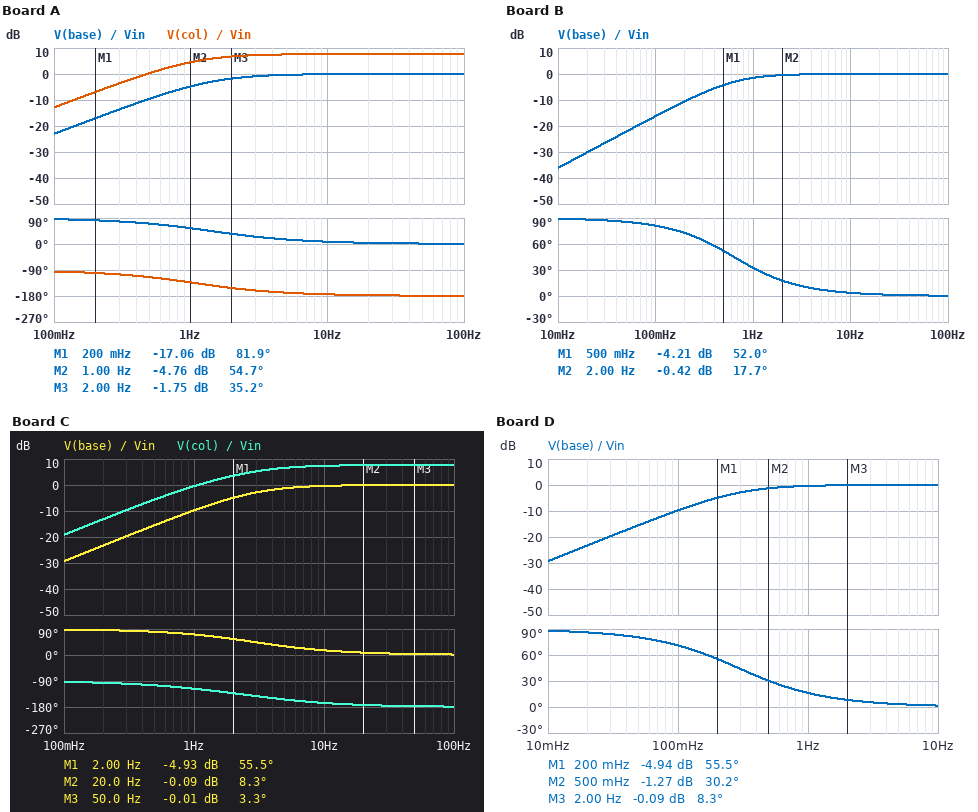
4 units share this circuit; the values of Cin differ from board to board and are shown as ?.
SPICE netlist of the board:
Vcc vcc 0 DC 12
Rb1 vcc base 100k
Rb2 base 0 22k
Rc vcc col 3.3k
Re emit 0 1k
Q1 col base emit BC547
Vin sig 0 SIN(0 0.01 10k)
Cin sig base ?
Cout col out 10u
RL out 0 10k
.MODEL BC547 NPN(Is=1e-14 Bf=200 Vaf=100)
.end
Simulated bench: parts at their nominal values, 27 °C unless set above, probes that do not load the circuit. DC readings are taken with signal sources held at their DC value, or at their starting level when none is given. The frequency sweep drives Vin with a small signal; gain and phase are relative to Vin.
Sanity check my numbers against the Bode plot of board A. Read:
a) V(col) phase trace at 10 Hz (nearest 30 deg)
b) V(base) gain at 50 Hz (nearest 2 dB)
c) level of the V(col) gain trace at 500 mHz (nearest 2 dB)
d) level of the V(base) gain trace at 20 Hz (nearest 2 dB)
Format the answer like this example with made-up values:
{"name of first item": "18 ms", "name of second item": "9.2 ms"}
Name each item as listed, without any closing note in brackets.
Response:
{"V(col) phase trace at 10 Hz": "-180 deg", "V(base) gain at 50 Hz": "0 dB", "level of the V(col) gain trace at 500 mHz": "0 dB", "level of the V(base) gain trace at 20 Hz": "0 dB"}
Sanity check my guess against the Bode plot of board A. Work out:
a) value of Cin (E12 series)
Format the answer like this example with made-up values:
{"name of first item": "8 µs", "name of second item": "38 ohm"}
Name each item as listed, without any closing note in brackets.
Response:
{"value of Cin": "6.8 µF"}
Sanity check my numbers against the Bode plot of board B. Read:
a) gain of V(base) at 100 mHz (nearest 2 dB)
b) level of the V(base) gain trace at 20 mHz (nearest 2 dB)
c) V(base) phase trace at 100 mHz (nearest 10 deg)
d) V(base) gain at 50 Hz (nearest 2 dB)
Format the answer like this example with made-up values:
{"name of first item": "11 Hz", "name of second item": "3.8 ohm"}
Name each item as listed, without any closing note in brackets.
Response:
{"gain of V(base) at 100 mHz": "-16 dB", "level of the V(base) gain trace at 20 mHz": "-30 dB", "V(base) phase trace at 100 mHz": "80 deg", "V(base) gain at 50 Hz": "0 dB"}
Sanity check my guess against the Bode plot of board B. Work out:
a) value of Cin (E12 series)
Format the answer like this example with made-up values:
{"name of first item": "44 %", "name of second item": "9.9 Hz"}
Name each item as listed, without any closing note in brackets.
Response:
{"value of Cin": "15 µF"}
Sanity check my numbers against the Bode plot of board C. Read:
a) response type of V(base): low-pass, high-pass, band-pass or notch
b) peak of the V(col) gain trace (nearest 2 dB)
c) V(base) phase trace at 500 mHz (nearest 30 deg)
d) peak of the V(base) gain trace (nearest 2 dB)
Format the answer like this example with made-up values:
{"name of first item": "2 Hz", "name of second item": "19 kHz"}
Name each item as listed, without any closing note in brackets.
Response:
{"response type of V(base): low-pass, high-pass, band-pass or notch": "high-pass", "peak of the V(col) gain trace": "8 dB", "V(base) phase trace at 500 mHz": "90 deg", "peak of the V(base) gain trace": "0 dB"}
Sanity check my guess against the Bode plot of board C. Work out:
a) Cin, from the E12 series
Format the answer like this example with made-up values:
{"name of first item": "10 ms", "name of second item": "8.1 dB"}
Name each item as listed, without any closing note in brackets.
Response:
{"Cin, from the E12 series": "3.3 µF"}
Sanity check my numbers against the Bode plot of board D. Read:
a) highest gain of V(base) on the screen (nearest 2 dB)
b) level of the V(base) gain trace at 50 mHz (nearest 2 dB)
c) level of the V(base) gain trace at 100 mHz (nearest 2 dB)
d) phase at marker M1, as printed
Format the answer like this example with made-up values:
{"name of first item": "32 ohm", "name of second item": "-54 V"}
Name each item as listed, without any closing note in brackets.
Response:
{"highest gain of V(base) on the screen": "0 dB", "level of the V(base) gain trace at 50 mHz": "-16 dB", "level of the V(base) gain trace at 100 mHz": "-10 dB", "phase at marker M1, as printed": "55.5 deg"}
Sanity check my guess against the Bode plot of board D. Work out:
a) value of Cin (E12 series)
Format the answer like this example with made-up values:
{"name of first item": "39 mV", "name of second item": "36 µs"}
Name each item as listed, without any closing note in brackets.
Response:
{"value of Cin": "33 µF"}
